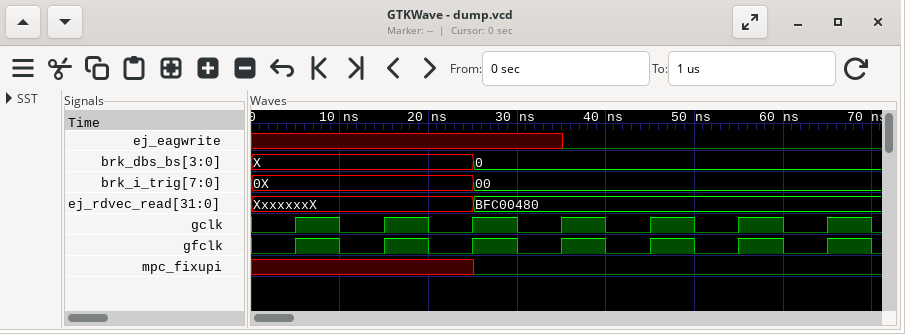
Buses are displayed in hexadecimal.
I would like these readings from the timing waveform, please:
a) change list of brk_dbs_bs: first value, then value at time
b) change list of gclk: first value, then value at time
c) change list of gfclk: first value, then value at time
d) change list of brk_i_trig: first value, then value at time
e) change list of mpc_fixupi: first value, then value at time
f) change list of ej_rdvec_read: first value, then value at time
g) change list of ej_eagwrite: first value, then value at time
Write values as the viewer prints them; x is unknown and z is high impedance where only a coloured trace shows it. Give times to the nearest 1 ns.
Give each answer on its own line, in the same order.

X, 0 at 25 ns
0, 1 at 5 ns, 0 at 10 ns, 1 at 15 ns, 0 at 20 ns, 1 at 25 ns, 0 at 30 ns, 1 at 35 ns, 0 at 40 ns, 1 at 45 ns, 0 at 50 ns, 1 at 55 ns, 0 at 60 ns, 1 at 65 ns, 0 at 70 ns
0, 1 at 5 ns, 0 at 10 ns, 1 at 15 ns, 0 at 20 ns, 1 at 25 ns, 0 at 30 ns, 1 at 35 ns, 0 at 40 ns, 1 at 45 ns, 0 at 50 ns, 1 at 55 ns, 0 at 60 ns, 1 at 65 ns, 0 at 70 ns
0X, 00 at 25 ns
x, 0 at 25 ns
XxxxxxxX, BFC00480 at 25 ns
x, 0 at 35 ns
